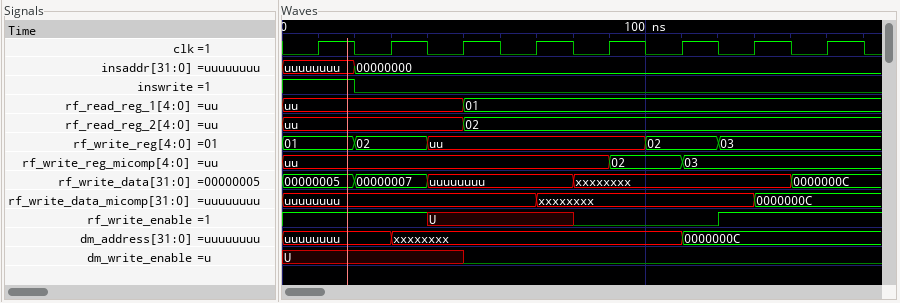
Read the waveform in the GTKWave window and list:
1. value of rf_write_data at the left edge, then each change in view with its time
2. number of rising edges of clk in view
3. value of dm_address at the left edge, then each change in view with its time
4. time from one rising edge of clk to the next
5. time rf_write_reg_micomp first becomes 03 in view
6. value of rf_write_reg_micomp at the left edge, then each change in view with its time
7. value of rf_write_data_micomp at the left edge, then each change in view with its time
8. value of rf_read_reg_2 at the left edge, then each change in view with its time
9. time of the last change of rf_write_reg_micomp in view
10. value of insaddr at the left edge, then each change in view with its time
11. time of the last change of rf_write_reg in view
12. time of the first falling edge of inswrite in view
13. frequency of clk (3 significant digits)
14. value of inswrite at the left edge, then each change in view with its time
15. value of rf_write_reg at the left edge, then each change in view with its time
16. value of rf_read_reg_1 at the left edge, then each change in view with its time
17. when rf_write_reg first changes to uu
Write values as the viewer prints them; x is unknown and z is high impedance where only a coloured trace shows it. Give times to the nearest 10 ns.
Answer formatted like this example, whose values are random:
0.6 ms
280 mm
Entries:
00000005, 00000007 at 20 ns, uuuuuuuu at 40 ns, xxxxxxxx at 80 ns, 0000000C at 140 ns
8
uuuuuuuu, xxxxxxxx at 30 ns, 0000000C at 110 ns
20 ns
110 ns
uu, 02 at 90 ns, 03 at 110 ns
uuuuuuuu, xxxxxxxx at 70 ns, 0000000C at 130 ns
uu, 02 at 50 ns
110 ns
uuuuuuuu, 00000000 at 20 ns
120 ns
20 ns
50.0 MHz
1, 0 at 20 ns
01, 02 at 20 ns, uu at 40 ns, 02 at 100 ns, 03 at 120 ns
uu, 01 at 50 ns
40 ns
